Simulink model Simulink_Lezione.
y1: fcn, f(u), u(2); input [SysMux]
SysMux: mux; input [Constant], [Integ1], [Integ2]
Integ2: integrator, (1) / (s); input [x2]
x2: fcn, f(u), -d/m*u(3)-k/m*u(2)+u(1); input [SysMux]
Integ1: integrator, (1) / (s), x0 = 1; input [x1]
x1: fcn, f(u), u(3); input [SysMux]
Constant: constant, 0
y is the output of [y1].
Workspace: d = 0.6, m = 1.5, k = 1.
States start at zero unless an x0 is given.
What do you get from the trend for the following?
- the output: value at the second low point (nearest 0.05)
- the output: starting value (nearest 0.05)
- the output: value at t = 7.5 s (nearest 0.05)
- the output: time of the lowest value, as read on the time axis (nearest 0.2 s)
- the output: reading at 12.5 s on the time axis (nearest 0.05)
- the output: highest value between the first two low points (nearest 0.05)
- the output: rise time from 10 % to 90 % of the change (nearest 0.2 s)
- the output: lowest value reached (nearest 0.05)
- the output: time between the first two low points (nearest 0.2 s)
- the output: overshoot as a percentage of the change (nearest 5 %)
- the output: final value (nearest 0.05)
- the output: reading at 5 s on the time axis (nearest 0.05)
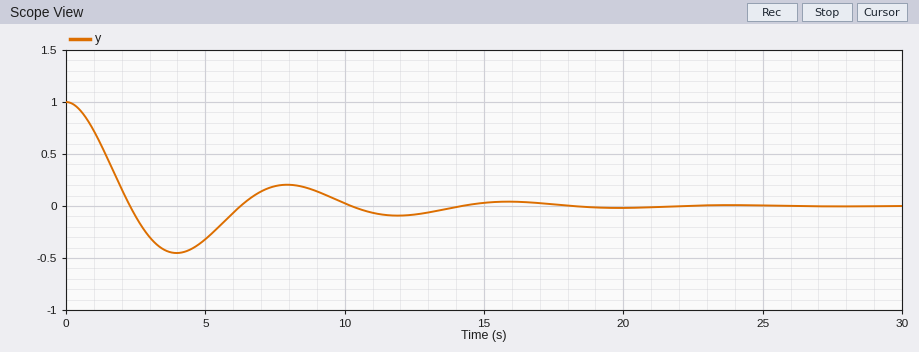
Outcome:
-0.10
1.00
0.20
4.0 s
-0.10
0.20
1.6 s
-0.45
8.0 s
45 %
0.00
-0.30
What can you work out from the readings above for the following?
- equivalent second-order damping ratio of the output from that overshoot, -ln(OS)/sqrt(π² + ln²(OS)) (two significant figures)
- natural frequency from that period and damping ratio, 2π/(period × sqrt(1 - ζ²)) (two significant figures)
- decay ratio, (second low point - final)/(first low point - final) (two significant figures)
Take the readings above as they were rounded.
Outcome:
0.25
0.81 rad/s
0.22
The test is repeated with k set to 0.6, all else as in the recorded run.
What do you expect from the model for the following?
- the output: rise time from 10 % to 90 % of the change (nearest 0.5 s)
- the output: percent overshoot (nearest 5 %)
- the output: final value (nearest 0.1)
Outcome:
2.0 s
35 %
0.0
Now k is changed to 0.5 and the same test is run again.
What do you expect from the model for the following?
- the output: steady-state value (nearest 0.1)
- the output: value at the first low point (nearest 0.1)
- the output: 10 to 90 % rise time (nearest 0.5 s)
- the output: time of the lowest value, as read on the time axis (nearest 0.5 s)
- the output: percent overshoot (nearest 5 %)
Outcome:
0.0
-0.3
2.5 s
6.0 s
30 %
